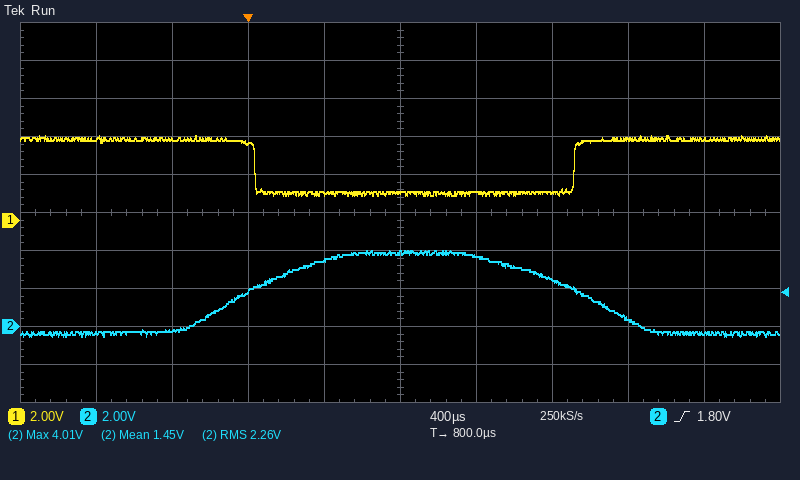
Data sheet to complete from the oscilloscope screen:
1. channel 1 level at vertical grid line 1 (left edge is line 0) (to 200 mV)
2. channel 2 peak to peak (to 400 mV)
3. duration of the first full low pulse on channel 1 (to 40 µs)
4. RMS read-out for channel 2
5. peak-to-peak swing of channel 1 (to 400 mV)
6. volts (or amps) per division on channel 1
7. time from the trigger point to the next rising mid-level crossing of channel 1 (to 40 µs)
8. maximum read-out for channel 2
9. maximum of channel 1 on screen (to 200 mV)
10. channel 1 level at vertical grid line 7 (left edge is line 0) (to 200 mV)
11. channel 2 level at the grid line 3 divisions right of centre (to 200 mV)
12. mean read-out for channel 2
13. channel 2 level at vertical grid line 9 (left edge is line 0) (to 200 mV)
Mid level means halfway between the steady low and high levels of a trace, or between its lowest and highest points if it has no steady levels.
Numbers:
4.4 V
4.4 V
1.68 ms
2.26 V
3.2 V
2 V
1.72 ms
4.01 V
4.4 V
1.4 V
400 mV
1.45 V
-400 mV
